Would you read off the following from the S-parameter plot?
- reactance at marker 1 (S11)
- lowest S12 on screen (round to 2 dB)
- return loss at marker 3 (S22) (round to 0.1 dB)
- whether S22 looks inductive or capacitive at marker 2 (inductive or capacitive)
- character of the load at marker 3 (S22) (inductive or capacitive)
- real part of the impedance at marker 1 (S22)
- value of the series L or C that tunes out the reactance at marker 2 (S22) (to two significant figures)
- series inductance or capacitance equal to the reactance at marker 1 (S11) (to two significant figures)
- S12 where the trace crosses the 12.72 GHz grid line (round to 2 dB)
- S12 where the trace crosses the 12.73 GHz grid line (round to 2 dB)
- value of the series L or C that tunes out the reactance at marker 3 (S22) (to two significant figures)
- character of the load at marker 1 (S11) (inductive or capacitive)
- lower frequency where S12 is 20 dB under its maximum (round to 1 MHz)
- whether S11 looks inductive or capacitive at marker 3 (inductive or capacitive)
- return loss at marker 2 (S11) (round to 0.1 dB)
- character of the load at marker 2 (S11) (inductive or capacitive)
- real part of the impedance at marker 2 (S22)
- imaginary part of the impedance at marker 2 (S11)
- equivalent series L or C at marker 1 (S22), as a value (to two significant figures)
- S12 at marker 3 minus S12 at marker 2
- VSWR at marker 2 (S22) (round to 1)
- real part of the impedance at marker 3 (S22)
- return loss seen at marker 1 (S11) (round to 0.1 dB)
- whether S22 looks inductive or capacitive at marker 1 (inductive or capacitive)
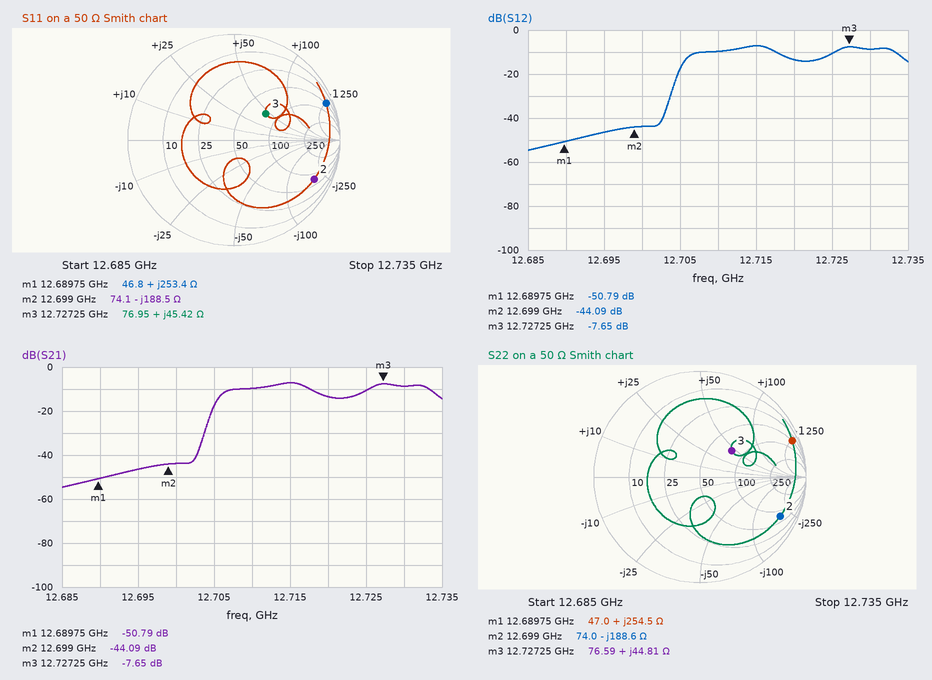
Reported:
+253.4 Ω
-54 dB
8.2 dB
capacitive
inductive
47.0 Ω
2.4 nH
3.2 nH
-14 dB
-8 dB
280 fF
inductive
12.704 GHz
inductive
1.5 dB
capacitive
74.0 Ω
-188.5 Ω
3.2 nH
36.44 dB
12
76.59 Ω
0.6 dB
inductive
